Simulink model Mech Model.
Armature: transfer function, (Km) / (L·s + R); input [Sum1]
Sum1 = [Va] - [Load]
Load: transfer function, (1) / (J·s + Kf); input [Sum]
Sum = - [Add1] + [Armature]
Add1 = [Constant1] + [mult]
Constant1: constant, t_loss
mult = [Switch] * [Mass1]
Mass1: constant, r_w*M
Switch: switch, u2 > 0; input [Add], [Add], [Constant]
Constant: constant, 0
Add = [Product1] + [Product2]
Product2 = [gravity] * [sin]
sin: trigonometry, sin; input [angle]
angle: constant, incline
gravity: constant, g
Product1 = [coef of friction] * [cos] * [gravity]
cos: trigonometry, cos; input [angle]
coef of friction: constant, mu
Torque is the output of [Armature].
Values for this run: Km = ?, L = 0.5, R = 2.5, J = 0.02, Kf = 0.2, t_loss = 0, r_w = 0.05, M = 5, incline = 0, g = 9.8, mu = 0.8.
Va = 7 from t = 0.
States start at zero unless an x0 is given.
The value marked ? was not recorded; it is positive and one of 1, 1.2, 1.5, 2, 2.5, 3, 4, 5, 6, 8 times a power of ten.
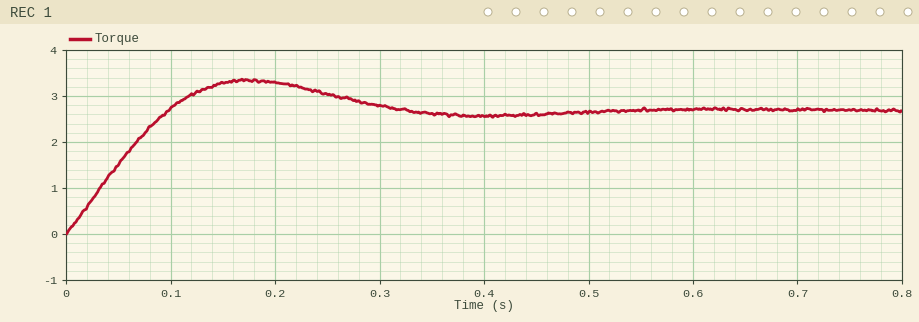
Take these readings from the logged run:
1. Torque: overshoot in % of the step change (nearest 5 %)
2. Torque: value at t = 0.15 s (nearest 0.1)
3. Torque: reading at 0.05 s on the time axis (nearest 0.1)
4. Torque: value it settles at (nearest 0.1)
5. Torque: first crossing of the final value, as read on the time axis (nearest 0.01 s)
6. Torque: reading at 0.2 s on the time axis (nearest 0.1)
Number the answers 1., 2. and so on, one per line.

1. 25 %
2. 3.3
3. 1.5
4. 2.7
5. 0.10 s
6. 3.3
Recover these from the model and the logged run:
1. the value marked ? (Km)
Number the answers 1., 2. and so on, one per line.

1. 2
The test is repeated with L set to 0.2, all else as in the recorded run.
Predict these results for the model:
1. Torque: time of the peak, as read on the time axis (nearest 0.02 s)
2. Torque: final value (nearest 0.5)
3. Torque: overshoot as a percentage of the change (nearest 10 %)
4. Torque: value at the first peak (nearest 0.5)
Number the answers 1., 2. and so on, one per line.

1. 0.10 s
2. 2.5
3. 40 %
4. 3.5
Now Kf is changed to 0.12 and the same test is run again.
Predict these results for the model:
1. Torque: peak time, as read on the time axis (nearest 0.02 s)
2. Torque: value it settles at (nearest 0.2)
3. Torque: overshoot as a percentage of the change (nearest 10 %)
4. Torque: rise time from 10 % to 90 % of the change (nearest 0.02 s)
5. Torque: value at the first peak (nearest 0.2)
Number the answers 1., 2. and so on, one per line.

1. 0.16 s
2. 2.4
3. 40 %
4. 0.06 s
5. 3.4
